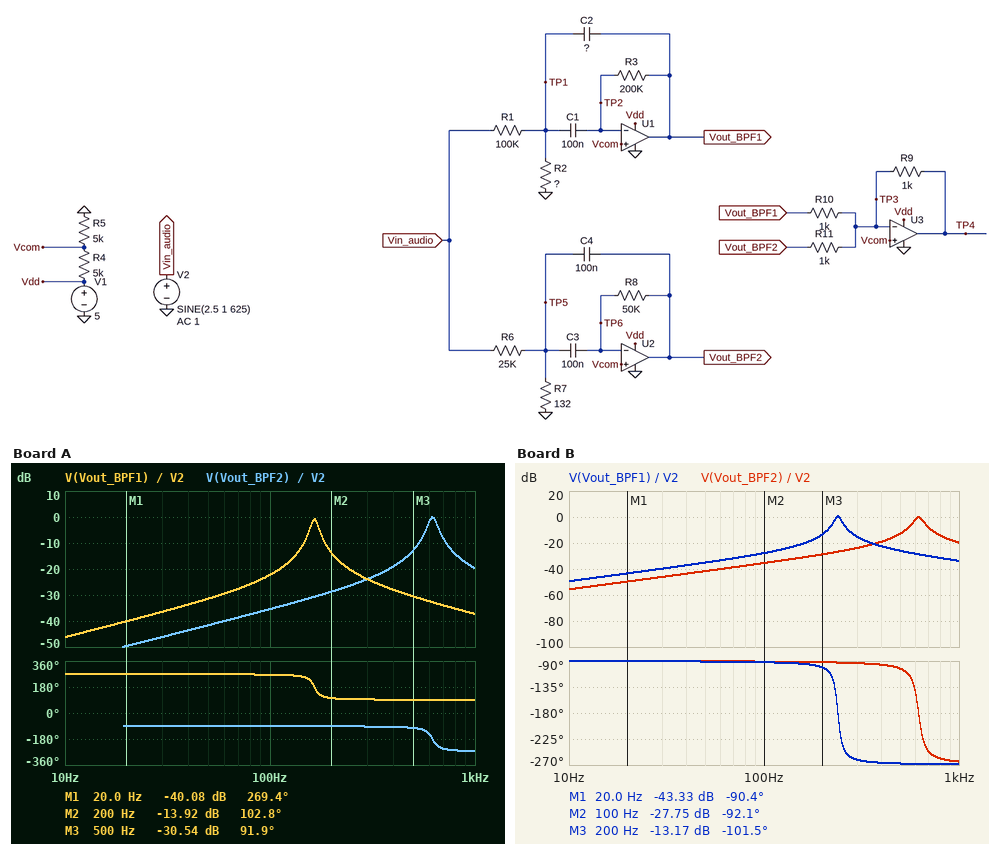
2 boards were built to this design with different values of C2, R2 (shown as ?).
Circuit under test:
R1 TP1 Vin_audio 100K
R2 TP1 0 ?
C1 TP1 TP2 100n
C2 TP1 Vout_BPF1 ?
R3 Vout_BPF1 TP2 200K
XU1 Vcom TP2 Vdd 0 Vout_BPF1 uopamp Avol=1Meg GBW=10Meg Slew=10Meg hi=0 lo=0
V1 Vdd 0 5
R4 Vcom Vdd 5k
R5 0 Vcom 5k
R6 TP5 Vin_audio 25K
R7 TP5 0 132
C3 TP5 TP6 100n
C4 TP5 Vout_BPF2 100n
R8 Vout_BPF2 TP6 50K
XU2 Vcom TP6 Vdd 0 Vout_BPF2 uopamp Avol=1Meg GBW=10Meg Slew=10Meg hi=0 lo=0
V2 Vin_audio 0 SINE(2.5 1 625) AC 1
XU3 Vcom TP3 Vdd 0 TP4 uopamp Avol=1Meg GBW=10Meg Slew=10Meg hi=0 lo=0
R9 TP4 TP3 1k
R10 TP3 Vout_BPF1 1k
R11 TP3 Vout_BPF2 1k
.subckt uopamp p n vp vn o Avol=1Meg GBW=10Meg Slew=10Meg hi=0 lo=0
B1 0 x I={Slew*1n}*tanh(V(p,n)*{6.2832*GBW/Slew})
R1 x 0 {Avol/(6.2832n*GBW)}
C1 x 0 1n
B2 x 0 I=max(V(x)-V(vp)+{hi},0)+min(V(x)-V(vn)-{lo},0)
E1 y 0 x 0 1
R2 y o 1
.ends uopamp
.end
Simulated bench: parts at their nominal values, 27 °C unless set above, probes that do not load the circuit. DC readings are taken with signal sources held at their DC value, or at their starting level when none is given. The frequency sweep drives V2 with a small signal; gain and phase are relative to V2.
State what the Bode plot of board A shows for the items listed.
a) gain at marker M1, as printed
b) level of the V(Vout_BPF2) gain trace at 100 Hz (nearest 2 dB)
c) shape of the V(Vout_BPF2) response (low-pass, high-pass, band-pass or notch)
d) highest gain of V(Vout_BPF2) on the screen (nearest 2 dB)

-40.08 dB
-36 dB
band-pass
0 dB
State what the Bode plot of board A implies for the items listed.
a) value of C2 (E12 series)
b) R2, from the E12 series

120 nF
390 Ω
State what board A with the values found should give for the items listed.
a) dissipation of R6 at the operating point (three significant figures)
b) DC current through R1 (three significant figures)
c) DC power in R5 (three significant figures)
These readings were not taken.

247 µW
24.9 µA
1.25 mW
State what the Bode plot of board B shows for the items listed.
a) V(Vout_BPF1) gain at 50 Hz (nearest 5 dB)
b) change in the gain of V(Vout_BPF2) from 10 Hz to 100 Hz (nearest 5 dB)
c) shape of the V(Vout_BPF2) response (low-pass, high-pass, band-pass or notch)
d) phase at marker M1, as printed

-35 dB
20 dB
band-pass
-90.4 deg
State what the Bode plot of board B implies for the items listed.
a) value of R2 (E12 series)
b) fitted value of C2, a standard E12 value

270 Ω
82 nF
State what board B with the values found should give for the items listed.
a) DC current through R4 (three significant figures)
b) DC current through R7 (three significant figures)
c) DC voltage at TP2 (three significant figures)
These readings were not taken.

500 µA
99.5 µA
2.50 V
